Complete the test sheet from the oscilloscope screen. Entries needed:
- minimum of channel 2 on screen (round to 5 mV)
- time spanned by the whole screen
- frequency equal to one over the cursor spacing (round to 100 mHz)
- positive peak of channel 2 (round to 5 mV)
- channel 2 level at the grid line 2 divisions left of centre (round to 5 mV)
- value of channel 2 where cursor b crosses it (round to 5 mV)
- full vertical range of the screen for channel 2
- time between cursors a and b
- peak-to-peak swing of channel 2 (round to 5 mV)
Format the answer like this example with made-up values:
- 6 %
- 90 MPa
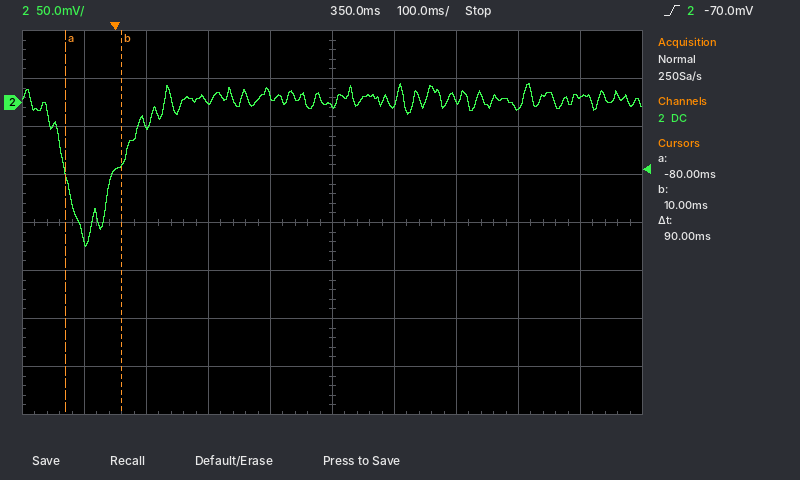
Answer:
- -150 mV
- 1 s
- 11.1 Hz
- 20 mV
- 0 mV
- -65 mV
- 400 mV
- 90 ms
- 170 mV
